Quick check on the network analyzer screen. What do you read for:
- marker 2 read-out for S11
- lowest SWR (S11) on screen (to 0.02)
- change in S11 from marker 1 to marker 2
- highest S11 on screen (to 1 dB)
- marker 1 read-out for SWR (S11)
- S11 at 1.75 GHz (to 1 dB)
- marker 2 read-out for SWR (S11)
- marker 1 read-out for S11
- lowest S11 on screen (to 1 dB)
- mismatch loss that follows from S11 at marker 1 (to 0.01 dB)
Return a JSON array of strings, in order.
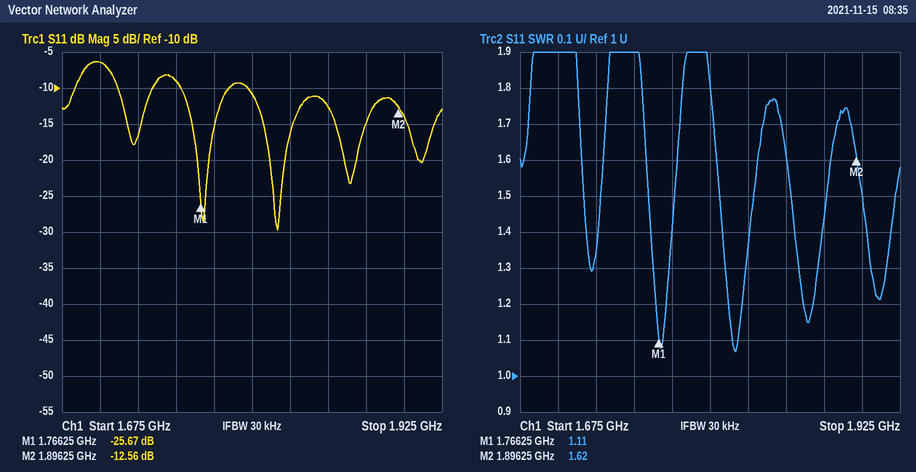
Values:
["-12.56 dB", "1.06", "13.11 dB", "-6 dB", "1.11", "-9 dB", "1.62", "-25.67 dB", "-30 dB", "0.01 dB"]
